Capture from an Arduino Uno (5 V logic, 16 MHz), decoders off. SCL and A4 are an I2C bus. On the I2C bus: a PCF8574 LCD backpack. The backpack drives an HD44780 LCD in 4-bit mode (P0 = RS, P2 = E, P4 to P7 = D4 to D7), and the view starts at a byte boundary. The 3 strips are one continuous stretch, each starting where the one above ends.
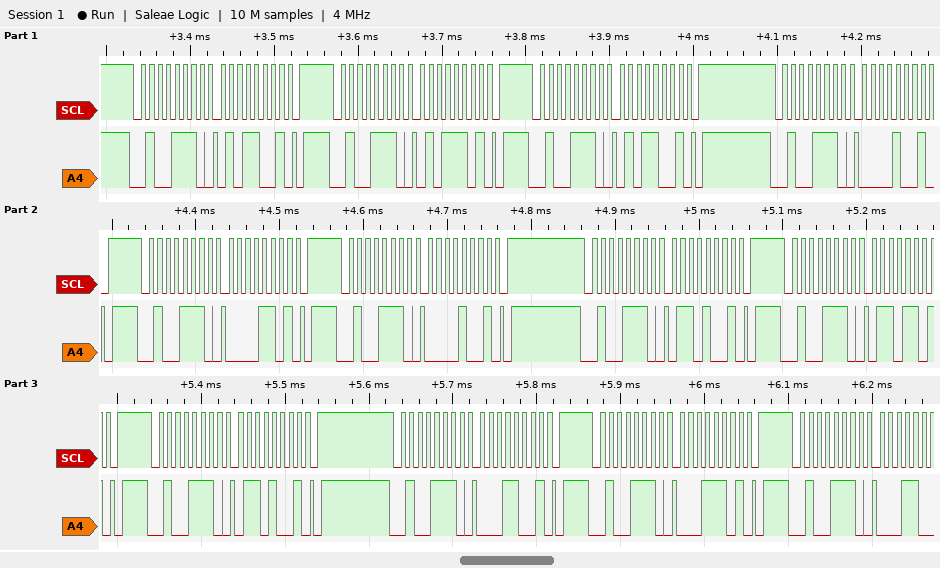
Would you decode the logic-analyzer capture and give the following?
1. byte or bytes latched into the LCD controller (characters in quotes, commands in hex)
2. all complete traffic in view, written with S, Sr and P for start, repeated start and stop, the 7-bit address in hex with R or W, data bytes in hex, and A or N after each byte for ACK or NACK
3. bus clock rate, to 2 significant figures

'P'
S 27W A 59 A P S 27W A 5D A P S 27W A 59 A P S 27W A 09 A P S 27W A 0D A P S 27W A 09 A P S 27W A 69 A P S 27W A 6D A P S 27W A 69 A P S 27W A 19 A P S 27W A 1D A P S 27W A
100 kHz
